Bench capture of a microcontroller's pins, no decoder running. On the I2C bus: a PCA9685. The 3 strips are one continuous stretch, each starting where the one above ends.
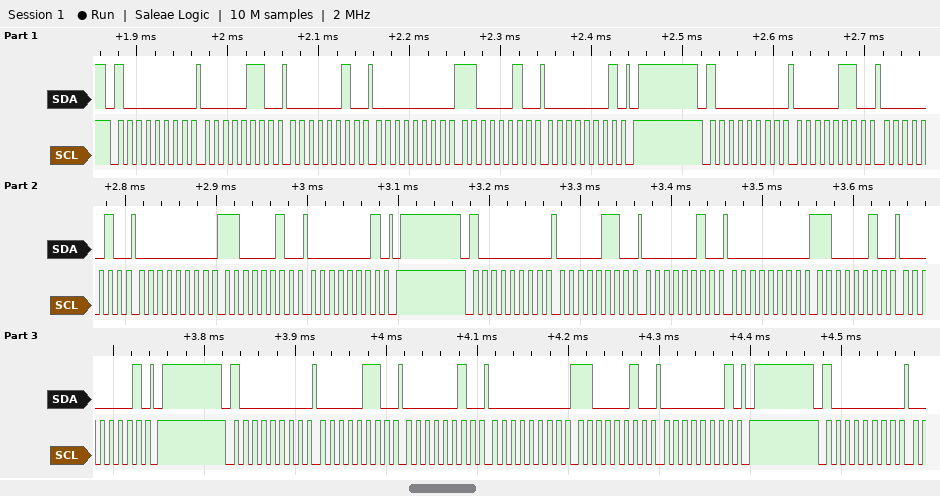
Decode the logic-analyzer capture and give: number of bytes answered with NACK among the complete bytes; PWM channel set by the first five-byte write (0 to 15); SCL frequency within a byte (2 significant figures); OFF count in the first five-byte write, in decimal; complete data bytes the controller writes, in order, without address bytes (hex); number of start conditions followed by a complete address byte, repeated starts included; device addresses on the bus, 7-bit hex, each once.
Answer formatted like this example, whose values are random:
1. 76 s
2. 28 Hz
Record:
1. 0
2. 0
3. 100 kHz
4. 450
5. 06 02 00 C2 01 06 02 00 C2 01 06 02 00 C2 01 06 02 00 C2 01
6. 5
7. 0x40
